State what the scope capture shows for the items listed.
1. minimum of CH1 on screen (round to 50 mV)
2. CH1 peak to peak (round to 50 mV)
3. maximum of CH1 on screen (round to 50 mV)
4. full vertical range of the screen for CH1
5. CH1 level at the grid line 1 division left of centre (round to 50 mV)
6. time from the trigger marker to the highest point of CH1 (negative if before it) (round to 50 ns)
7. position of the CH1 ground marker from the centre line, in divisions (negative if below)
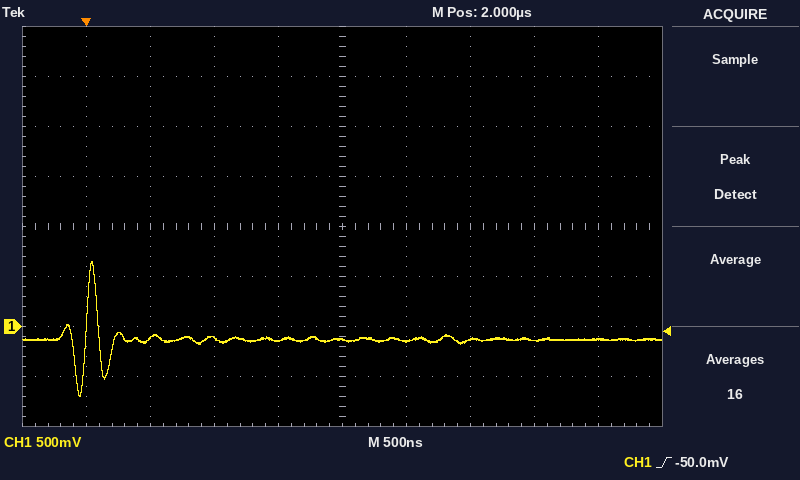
-700 mV
1.35 V
650 mV
4 V
-150 mV
+50 ns
-2.0 div
